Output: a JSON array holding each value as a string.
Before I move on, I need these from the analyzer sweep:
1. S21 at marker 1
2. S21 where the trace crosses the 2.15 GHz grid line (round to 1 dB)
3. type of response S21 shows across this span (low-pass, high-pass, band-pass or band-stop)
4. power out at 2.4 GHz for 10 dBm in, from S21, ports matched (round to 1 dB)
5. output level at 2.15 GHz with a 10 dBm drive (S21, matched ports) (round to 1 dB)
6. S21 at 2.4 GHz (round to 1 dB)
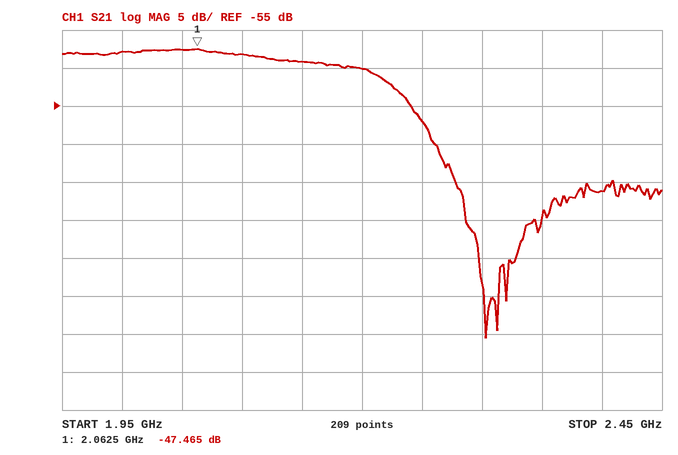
["-47.465 dB", "-49 dB", "low-pass", "-56 dBm", "-39 dBm", "-66 dB"]
